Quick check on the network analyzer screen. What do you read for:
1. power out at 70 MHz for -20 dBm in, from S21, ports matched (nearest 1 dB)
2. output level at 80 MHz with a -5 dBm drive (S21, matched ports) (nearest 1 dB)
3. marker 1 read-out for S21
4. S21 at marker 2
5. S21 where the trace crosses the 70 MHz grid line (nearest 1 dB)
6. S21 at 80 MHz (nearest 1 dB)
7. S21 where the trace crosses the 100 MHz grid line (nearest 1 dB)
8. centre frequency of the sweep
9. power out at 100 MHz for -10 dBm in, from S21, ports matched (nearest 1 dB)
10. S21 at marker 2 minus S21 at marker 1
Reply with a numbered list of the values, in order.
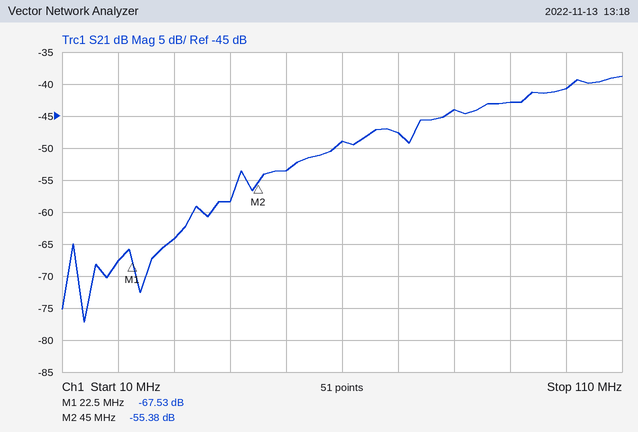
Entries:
1. -68 dBm
2. -49 dBm
3. -67.53 dB
4. -55.38 dB
5. -48 dB
6. -44 dB
7. -41 dB
8. 60 MHz
9. -51 dBm
10. 12.15 dB
